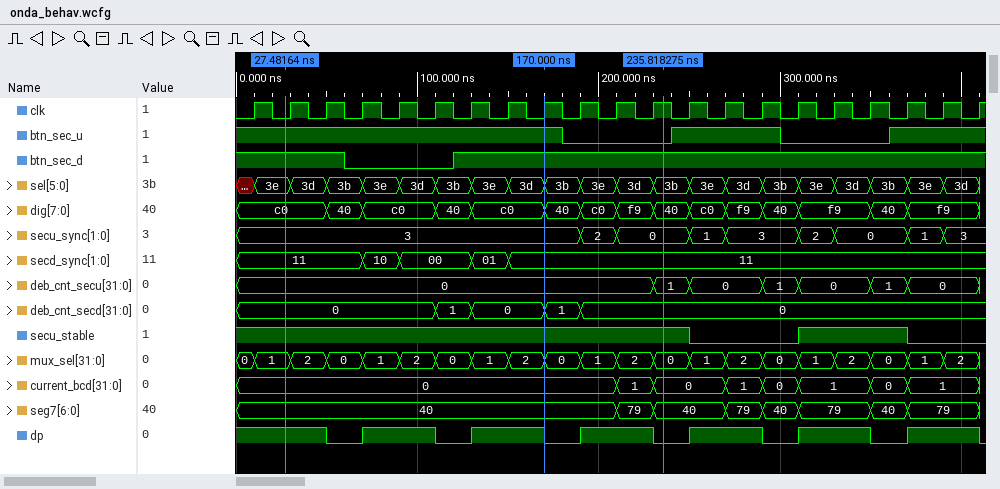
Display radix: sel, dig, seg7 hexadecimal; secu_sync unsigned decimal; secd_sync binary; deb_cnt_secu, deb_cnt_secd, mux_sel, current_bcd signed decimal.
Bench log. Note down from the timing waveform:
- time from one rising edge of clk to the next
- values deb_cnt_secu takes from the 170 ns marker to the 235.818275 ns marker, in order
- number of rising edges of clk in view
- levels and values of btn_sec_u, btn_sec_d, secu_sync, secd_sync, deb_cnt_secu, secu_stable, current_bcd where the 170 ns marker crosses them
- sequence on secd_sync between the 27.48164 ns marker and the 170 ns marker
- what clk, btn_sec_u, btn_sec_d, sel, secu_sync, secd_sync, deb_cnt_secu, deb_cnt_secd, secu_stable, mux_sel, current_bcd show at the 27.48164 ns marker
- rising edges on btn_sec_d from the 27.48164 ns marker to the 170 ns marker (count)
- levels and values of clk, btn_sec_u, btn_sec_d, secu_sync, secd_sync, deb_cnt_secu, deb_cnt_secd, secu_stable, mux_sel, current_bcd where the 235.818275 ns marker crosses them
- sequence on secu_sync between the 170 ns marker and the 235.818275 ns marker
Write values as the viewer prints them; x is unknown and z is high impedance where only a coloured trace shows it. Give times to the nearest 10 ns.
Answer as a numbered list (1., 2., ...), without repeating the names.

1. 20 ns
2. 0, 1
3. 21
4. btn_sec_u=1, btn_sec_d=1, secu_sync=3, secd_sync=11, deb_cnt_secu=0, secu_stable=1, current_bcd=0
5. 11, 10, 00, 01, 11
6. clk=0, btn_sec_u=1, btn_sec_d=1, sel=3e, secu_sync=3, secd_sync=11, deb_cnt_secu=0, deb_cnt_secd=0, secu_stable=1, mux_sel=1, current_bcd=0
7. 1
8. clk=1, btn_sec_u=0, btn_sec_d=1, secu_sync=0, secd_sync=11, deb_cnt_secu=1, deb_cnt_secd=0, secu_stable=1, mux_sel=0, current_bcd=0
9. 3, 2, 0
